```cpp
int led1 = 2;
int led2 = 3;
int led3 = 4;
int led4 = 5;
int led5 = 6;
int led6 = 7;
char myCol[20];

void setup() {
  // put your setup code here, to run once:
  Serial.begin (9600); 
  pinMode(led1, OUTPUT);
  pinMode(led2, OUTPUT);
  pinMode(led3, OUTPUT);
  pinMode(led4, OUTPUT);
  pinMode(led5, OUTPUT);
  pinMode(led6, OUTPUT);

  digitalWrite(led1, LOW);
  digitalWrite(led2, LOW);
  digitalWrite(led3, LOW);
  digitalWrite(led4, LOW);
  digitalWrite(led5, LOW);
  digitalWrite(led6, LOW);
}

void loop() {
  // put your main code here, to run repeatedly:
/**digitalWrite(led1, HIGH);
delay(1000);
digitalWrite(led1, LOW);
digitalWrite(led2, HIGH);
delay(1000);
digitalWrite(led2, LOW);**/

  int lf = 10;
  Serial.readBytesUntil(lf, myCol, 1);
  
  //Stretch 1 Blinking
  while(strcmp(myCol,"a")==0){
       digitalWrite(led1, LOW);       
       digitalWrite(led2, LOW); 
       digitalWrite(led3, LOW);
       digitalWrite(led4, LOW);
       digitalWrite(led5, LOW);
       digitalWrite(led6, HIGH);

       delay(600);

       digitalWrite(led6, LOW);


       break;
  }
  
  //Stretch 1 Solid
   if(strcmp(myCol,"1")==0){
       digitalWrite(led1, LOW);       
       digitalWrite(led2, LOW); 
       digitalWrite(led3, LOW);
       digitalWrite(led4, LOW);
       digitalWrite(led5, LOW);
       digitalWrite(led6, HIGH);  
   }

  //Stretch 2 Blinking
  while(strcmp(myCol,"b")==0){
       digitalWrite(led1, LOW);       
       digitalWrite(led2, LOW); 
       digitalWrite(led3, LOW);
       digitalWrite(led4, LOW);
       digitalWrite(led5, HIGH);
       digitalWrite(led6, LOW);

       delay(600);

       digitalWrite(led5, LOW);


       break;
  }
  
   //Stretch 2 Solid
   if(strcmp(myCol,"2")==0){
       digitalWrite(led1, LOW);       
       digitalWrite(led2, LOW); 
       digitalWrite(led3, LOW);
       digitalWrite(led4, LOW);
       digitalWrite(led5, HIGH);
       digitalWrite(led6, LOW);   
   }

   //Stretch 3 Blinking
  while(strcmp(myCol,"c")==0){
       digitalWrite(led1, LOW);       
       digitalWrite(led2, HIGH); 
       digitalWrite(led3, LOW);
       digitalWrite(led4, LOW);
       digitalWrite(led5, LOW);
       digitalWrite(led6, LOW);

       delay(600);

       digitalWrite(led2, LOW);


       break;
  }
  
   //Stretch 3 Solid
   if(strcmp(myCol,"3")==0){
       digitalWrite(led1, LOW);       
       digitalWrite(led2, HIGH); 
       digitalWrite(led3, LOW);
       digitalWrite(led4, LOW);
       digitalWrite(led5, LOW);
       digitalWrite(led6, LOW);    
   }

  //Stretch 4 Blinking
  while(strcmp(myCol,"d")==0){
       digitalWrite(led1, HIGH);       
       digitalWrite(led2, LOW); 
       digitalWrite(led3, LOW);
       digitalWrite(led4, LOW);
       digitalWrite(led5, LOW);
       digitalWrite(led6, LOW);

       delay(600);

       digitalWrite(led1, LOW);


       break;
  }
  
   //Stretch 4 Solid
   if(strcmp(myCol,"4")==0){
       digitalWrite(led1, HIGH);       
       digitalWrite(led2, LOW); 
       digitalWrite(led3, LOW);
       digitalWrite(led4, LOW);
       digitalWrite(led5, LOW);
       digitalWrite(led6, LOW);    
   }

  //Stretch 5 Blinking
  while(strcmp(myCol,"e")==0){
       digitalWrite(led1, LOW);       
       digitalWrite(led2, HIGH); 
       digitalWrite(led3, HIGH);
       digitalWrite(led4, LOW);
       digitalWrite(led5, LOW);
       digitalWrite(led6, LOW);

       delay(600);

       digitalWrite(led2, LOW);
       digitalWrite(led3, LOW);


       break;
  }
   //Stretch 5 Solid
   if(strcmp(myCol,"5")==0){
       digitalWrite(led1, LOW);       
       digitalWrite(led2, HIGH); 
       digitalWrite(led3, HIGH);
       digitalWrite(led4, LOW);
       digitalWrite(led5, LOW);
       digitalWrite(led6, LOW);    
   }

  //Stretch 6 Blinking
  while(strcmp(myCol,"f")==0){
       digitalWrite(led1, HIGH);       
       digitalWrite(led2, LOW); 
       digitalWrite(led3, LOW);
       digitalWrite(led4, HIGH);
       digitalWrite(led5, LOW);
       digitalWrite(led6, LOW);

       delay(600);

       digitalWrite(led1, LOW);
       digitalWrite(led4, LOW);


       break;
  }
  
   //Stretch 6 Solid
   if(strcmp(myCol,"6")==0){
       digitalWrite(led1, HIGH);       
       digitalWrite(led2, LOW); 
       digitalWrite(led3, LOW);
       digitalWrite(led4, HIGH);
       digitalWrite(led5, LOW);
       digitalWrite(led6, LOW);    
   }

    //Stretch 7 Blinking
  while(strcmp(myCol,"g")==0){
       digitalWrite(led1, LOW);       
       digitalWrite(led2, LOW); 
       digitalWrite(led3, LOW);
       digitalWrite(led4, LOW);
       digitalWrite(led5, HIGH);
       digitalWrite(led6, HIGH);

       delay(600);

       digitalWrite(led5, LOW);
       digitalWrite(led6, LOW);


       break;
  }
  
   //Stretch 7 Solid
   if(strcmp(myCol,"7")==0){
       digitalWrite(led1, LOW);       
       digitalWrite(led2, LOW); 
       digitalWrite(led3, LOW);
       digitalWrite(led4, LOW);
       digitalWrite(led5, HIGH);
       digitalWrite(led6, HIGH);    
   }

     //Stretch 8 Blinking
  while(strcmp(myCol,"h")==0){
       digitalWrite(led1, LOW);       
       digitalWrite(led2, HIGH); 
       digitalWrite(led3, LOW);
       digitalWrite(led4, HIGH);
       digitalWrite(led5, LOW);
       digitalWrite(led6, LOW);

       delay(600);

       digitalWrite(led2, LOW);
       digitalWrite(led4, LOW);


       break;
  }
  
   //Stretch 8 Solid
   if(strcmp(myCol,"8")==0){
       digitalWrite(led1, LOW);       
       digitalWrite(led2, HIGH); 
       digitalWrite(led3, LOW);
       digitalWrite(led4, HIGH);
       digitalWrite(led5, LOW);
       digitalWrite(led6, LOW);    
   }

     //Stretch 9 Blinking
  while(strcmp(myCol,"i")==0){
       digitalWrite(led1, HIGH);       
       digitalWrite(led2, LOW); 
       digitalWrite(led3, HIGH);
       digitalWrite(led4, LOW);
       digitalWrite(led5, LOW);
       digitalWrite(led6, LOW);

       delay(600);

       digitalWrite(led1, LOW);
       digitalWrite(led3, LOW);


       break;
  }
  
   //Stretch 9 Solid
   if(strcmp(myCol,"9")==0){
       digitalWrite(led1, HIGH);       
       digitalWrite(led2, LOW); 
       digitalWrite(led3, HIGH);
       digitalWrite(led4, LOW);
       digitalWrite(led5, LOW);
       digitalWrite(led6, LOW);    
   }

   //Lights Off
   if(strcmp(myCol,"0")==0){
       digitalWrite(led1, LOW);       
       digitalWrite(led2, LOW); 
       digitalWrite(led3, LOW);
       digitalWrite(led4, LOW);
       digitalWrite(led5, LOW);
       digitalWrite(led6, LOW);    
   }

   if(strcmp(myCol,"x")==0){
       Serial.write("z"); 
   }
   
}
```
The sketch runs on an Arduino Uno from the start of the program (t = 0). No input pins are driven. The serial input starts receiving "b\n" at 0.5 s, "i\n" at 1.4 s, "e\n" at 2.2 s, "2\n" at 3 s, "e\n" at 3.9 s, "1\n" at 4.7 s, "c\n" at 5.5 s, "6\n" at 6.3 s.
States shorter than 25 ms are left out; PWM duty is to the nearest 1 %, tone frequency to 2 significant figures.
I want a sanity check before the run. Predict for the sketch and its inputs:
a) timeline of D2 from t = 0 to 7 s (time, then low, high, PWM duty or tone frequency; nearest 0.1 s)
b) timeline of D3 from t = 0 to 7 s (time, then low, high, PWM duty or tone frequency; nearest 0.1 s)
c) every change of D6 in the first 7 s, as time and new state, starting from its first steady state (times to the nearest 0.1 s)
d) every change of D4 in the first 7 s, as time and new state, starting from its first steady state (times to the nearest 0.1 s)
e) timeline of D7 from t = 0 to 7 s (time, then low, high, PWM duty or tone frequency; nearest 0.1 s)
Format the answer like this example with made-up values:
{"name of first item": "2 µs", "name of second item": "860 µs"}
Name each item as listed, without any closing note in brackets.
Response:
{"timeline of D2 from t = 0 to 7 s": "0 s low; 1.7 s high; 2.9 s low; 6.7 s high", "timeline of D3 from t = 0 to 7 s": "0 s low; 2.9 s high; 5.3 s low; 5.5 s high; 6.7 s low", "every change of D6 in the first 7 s, as time and new state, starting from its first steady state": "0 s low; 0.5 s high; 1.7 s low", "every change of D4 in the first 7 s, as time and new state, starting from its first steady state": "0 s low; 1.7 s high; 5.3 s low", "timeline of D7 from t = 0 to 7 s": "0 s low; 5.3 s high; 5.5 s low"}
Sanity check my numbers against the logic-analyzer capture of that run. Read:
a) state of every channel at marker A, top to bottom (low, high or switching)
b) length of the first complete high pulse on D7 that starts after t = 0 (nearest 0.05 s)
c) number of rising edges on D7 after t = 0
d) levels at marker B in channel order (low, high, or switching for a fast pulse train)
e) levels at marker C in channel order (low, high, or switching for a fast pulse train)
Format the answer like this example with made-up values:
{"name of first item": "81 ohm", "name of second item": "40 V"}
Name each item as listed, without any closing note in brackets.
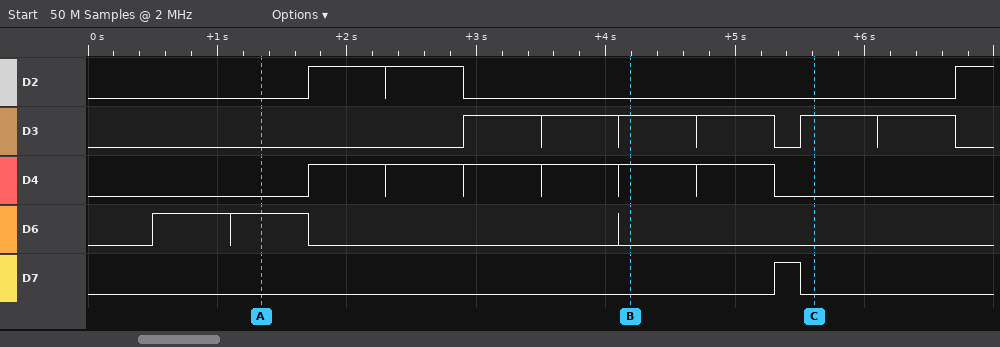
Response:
{"state of every channel at marker A, top to bottom": "D2 low, D3 low, D4 low, D6 high, D7 low", "length of the first complete high pulse on D7 that starts after t = 0": "0.20 s", "number of rising edges on D7 after t = 0": "1", "levels at marker B in channel order": "D2 low, D3 high, D4 high, D6 low, D7 low", "levels at marker C in channel order": "D2 low, D3 high, D4 low, D6 low, D7 low"}
